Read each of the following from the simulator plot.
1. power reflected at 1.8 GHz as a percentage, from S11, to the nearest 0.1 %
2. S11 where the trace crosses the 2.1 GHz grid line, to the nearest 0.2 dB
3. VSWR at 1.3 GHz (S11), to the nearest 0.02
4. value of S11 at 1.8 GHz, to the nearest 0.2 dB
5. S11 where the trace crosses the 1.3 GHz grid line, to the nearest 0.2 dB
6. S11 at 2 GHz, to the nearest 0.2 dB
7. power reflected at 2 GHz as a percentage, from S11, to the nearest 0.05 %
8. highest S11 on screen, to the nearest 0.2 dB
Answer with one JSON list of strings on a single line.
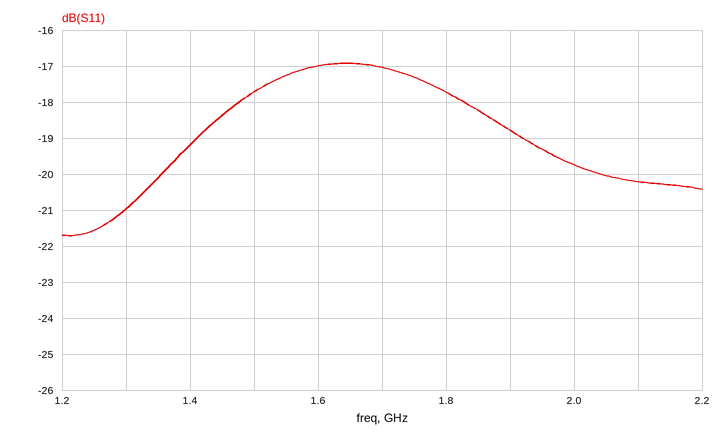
["1.7 %", "-20.2 dB", "1.20", "-17.8 dB", "-21.0 dB", "-19.8 dB", "1.05 %", "-17.0 dB"]
